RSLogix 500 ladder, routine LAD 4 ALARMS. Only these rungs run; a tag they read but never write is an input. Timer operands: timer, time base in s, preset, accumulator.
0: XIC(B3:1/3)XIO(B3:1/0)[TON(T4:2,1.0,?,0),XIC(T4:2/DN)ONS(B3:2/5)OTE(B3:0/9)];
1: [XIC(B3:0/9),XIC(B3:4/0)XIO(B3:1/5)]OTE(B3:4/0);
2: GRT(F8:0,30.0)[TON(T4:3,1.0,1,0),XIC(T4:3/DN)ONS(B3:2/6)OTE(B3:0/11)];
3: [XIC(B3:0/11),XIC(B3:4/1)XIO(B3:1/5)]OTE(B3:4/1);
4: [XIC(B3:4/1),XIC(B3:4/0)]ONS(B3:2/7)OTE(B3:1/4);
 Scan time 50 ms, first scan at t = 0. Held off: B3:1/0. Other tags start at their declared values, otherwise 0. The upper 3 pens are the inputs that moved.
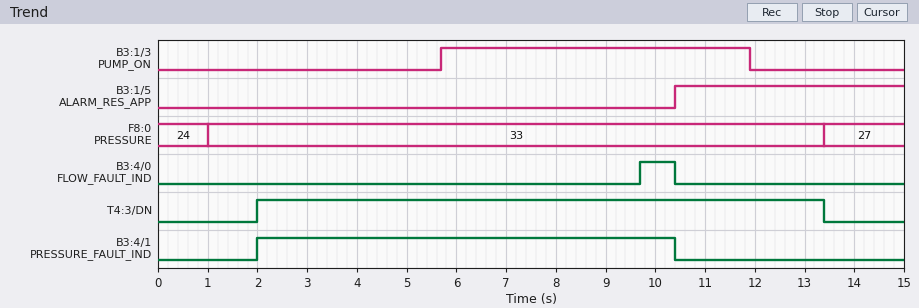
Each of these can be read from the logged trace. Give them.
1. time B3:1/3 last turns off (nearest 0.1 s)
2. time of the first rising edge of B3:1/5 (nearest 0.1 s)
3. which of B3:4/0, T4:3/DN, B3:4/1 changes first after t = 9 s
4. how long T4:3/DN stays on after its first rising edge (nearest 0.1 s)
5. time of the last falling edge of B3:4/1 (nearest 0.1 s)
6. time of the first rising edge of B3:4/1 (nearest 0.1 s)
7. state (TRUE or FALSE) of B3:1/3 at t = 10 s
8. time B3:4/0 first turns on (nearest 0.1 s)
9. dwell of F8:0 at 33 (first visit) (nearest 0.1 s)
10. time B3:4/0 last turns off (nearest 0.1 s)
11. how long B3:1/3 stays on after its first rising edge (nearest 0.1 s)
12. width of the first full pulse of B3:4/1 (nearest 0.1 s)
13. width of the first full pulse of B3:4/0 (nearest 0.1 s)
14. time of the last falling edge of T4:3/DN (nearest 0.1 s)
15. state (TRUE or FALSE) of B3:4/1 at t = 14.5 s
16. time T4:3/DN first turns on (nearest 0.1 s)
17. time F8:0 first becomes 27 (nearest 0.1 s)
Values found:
11.9 s
10.4 s
B3:4/0
11.4 s
10.4 s
2.0 s
TRUE
9.7 s
12.4 s
10.4 s
6.2 s
8.4 s
0.7 s
13.4 s
FALSE
2.0 s
13.4 s
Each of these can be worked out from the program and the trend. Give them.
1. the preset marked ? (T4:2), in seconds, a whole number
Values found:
4 s
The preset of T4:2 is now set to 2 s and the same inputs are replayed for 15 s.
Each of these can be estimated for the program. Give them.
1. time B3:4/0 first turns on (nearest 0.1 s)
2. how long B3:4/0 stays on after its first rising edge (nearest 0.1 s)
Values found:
7.7 s
2.7 s
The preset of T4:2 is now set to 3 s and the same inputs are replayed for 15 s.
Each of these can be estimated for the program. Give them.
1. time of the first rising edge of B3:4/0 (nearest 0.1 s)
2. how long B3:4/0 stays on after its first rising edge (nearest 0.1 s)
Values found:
8.7 s
1.7 s
